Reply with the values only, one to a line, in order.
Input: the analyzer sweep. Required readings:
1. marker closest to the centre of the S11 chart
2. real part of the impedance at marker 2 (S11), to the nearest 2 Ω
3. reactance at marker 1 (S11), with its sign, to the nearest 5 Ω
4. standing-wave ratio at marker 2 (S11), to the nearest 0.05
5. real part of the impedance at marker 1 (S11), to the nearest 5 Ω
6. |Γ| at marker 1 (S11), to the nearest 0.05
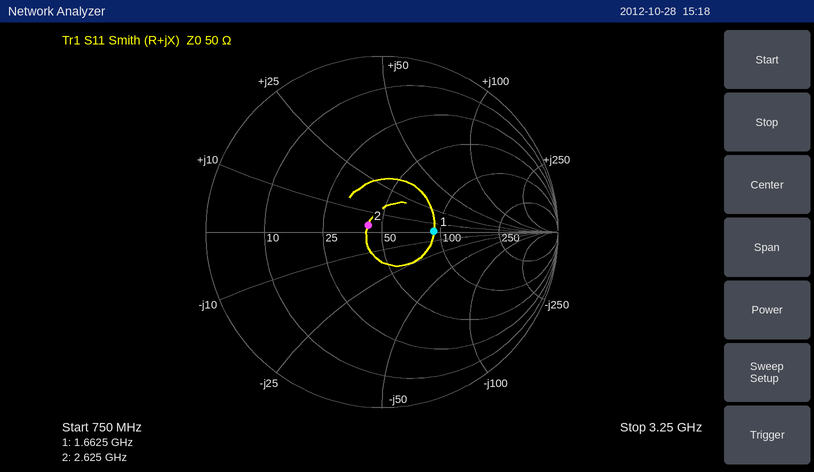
marker 2
42 Ω
0 Ω
1.20
90 Ω
0.30
